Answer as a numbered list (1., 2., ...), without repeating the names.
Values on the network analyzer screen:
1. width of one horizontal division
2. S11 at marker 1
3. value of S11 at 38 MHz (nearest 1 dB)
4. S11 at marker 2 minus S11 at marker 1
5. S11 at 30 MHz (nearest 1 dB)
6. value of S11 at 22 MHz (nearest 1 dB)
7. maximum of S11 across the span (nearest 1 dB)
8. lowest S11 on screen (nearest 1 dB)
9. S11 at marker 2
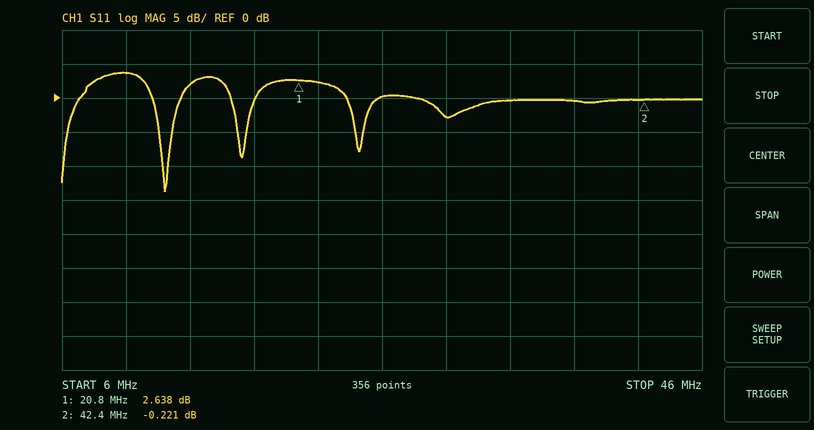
1. 4 MHz
2. 2.638 dB
3. 0 dB
4. -2.859 dB
5. -3 dB
6. 2 dB
7. 4 dB
8. -14 dB
9. -0.221 dB
